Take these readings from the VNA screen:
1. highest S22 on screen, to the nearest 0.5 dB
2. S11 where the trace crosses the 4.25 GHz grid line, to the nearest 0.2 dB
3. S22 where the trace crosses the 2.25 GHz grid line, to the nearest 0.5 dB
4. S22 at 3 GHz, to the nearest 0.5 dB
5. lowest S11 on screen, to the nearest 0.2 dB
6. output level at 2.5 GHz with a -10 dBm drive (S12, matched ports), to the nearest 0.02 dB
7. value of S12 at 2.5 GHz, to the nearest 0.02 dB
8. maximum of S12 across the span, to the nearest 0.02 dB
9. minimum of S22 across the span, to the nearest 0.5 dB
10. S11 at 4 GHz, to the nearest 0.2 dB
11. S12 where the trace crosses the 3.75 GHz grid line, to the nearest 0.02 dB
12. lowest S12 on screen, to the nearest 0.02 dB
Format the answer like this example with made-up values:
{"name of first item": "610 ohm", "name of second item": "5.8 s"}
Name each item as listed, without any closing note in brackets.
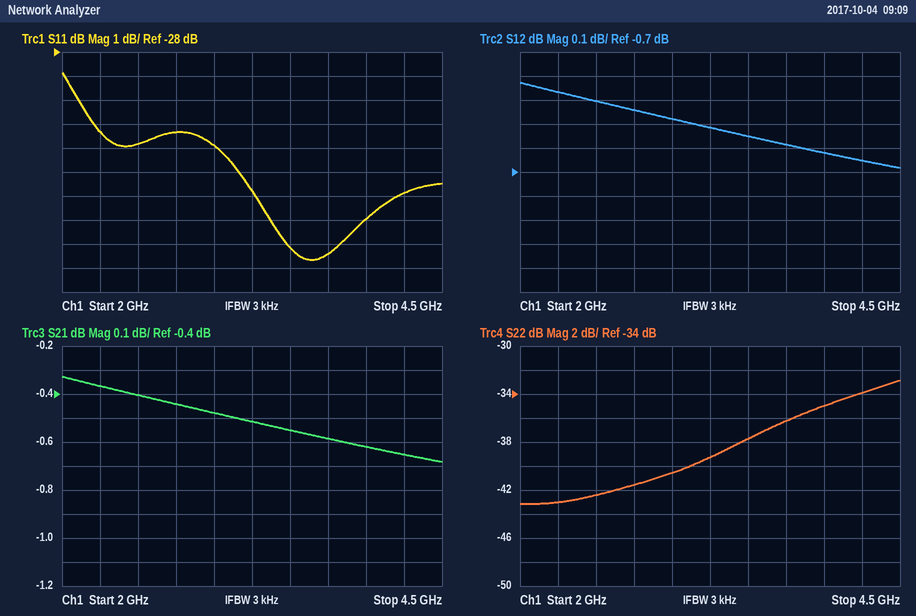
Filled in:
{"highest S22 on screen, to the nearest 0.5 dB": "-33.0 dB", "S11 where the trace crosses the 4.25 GHz grid line, to the nearest 0.2 dB": "-33.8 dB", "S22 where the trace crosses the 2.25 GHz grid line, to the nearest 0.5 dB": "-43.0 dB", "S22 at 3 GHz, to the nearest 0.5 dB": "-40.5 dB", "lowest S11 on screen, to the nearest 0.2 dB": "-36.6 dB", "output level at 2.5 GHz with a -10 dBm drive (S12, matched ports), to the nearest 0.02 dB": "-10.40 dBm", "value of S12 at 2.5 GHz, to the nearest 0.02 dB": "-0.40 dB", "maximum of S12 across the span, to the nearest 0.02 dB": "-0.32 dB", "minimum of S22 across the span, to the nearest 0.5 dB": "-43.0 dB", "S11 at 4 GHz, to the nearest 0.2 dB": "-35.0 dB", "S12 where the trace crosses the 3.75 GHz grid line, to the nearest 0.02 dB": "-0.58 dB", "lowest S12 on screen, to the nearest 0.02 dB": "-0.68 dB"}
